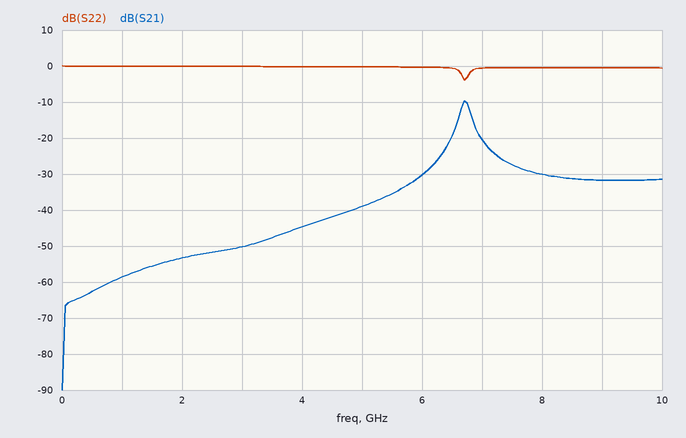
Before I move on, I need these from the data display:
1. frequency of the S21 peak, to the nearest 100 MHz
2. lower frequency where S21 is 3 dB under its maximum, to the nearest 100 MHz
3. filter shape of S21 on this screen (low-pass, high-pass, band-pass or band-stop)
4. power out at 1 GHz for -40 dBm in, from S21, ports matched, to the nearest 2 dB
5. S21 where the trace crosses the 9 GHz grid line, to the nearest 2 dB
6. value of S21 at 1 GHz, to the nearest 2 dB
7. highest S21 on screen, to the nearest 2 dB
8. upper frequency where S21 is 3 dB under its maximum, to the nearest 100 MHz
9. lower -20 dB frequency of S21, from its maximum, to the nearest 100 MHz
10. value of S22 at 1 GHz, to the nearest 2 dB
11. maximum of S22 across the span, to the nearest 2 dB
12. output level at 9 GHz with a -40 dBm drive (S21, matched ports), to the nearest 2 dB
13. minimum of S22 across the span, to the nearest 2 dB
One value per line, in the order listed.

6.7 GHz
6.6 GHz
band-pass
-98 dBm
-32 dB
-58 dB
-10 dB
6.8 GHz
6.0 GHz
0 dB
0 dB
-72 dBm
-4 dB
